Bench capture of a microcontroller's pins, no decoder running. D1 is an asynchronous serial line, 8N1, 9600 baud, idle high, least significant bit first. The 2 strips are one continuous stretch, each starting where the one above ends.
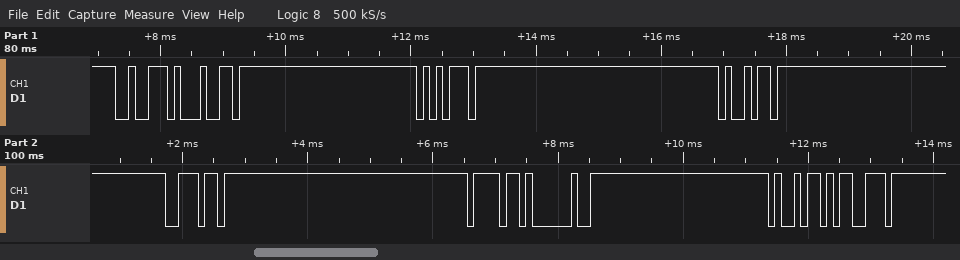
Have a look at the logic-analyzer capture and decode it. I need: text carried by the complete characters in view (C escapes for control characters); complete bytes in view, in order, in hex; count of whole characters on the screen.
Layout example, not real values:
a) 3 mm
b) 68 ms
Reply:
a) "rduino is"
b) 0x72 0x64 0x75 0x69 0x6E 0x6F 0x20 0x69 0x73
c) 9
